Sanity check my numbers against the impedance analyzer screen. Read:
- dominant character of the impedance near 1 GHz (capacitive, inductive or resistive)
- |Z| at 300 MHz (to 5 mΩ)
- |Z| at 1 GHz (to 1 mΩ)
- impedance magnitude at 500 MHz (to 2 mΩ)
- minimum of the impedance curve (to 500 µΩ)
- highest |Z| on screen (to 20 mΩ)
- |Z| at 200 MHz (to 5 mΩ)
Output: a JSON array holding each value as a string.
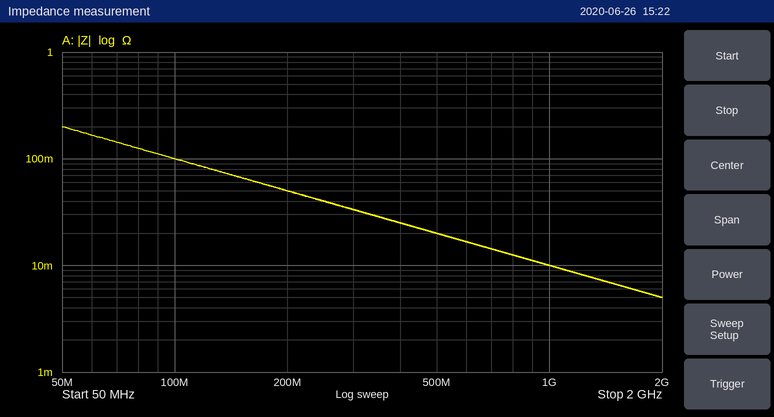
["capacitive", "35 mΩ", "10 mΩ", "20 mΩ", "5.0 mΩ", "200 mΩ", "50 mΩ"]
